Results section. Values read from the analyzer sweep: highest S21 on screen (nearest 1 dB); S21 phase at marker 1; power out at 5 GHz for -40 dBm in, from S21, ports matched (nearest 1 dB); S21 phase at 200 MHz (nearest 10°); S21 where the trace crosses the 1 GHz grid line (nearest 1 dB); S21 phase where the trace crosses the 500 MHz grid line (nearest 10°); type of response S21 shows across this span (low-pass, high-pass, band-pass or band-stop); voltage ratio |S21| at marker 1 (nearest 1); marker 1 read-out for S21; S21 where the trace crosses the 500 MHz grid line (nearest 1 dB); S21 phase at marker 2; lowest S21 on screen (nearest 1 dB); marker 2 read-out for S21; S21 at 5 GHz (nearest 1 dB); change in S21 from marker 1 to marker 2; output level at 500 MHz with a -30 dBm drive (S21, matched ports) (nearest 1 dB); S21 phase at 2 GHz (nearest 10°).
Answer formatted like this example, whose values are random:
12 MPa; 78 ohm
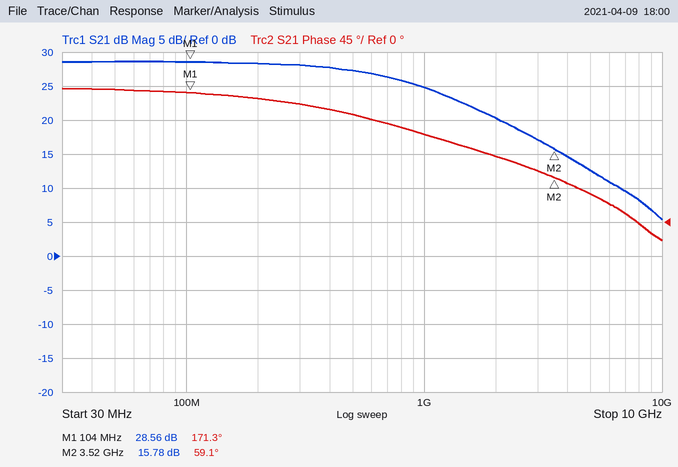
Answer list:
29 dB; 171.3°; -27 dBm; 160°; 25 dB; 140°; low-pass; 27; 28.56 dB; 27 dB; 59.1°; 5 dB; 15.78 dB; 13 dB; -12.78 dB; -3 dBm; 90°
